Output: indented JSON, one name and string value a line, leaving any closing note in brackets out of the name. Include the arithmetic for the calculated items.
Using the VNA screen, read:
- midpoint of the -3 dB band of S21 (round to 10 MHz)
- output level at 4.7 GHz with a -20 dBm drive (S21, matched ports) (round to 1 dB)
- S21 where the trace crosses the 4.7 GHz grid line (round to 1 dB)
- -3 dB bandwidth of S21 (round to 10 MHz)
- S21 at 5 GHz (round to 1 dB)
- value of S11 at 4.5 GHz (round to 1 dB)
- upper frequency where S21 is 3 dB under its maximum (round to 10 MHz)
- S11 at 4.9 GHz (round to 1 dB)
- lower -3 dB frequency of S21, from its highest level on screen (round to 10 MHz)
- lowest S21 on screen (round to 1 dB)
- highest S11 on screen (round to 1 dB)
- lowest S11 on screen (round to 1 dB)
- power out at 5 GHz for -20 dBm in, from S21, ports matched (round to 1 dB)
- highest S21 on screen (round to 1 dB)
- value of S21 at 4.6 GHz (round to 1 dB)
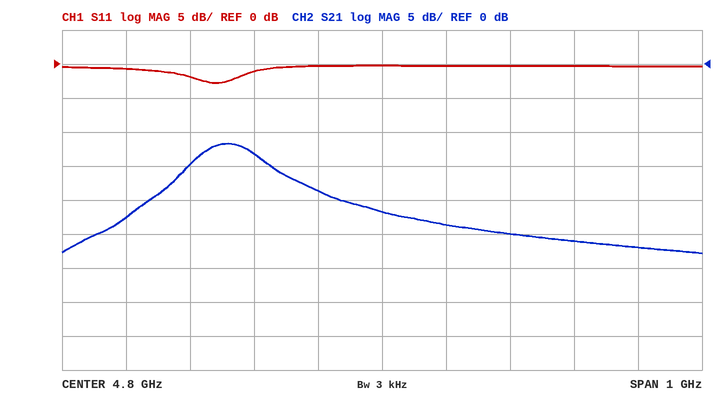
{
  "midpoint of the -3 dB band of S21": "4.56 GHz",
  "output level at 4.7 GHz with a -20 dBm drive (S21, matched ports)": "-20 dBm + (-19 dB) = -39 dBm",
  "S21 where the trace crosses the 4.7 GHz grid line": "-19 dB",
  "-3 dB bandwidth of S21": "4.62 GHz − 4.50 GHz = 120 MHz",
  "S21 at 5 GHz": "-25 dB",
  "value of S11 at 4.5 GHz": "-2 dB",
  "upper frequency where S21 is 3 dB under its maximum": "4.62 GHz",
  "S11 at 4.9 GHz": "0 dB",
  "lower -3 dB frequency of S21, from its highest level on screen": "4.50 GHz",
  "lowest S21 on screen": "-28 dB",
  "highest S11 on screen": "0 dB",
  "lowest S11 on screen": "-3 dB",
  "power out at 5 GHz for -20 dBm in, from S21, ports matched": "-20 dBm + (-25 dB) = -45 dBm",
  "highest S21 on screen": "-12 dB",
  "value of S21 at 4.6 GHz": "-13 dB"
}
